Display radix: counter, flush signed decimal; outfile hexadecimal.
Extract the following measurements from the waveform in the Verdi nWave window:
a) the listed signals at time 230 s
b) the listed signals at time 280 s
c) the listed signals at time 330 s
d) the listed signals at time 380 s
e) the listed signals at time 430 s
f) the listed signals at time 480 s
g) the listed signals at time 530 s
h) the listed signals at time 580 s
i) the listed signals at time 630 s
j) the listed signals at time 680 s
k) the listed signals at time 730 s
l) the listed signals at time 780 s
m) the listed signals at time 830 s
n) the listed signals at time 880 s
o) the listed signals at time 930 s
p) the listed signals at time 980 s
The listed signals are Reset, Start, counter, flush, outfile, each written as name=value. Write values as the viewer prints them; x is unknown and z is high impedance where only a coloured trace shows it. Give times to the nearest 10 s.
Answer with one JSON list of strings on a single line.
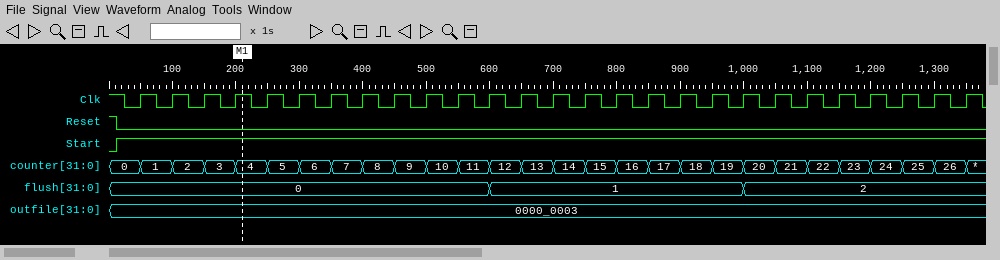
["Reset=0, Start=1, counter=4, flush=0, outfile=0000_0003", "Reset=0, Start=1, counter=5, flush=0, outfile=0000_0003", "Reset=0, Start=1, counter=6, flush=0, outfile=0000_0003", "Reset=0, Start=1, counter=7, flush=0, outfile=0000_0003", "Reset=0, Start=1, counter=8, flush=0, outfile=0000_0003", "Reset=0, Start=1, counter=9, flush=0, outfile=0000_0003", "Reset=0, Start=1, counter=10, flush=0, outfile=0000_0003", "Reset=0, Start=1, counter=11, flush=0, outfile=0000_0003", "Reset=0, Start=1, counter=12, flush=1, outfile=0000_0003", "Reset=0, Start=1, counter=13, flush=1, outfile=0000_0003", "Reset=0, Start=1, counter=14, flush=1, outfile=0000_0003", "Reset=0, Start=1, counter=15, flush=1, outfile=0000_0003", "Reset=0, Start=1, counter=16, flush=1, outfile=0000_0003", "Reset=0, Start=1, counter=17, flush=1, outfile=0000_0003", "Reset=0, Start=1, counter=18, flush=1, outfile=0000_0003", "Reset=0, Start=1, counter=19, flush=1, outfile=0000_0003"]
